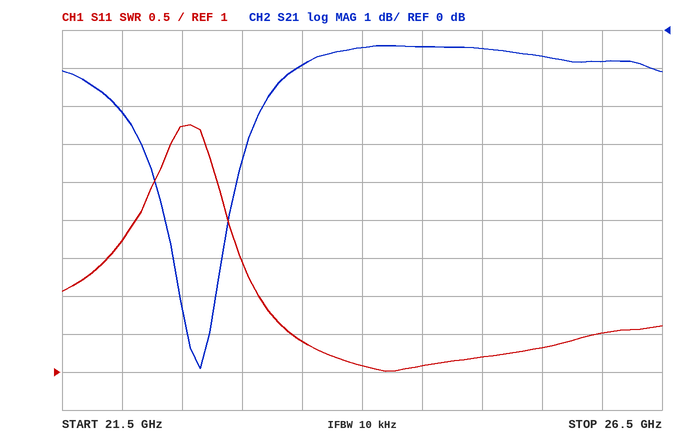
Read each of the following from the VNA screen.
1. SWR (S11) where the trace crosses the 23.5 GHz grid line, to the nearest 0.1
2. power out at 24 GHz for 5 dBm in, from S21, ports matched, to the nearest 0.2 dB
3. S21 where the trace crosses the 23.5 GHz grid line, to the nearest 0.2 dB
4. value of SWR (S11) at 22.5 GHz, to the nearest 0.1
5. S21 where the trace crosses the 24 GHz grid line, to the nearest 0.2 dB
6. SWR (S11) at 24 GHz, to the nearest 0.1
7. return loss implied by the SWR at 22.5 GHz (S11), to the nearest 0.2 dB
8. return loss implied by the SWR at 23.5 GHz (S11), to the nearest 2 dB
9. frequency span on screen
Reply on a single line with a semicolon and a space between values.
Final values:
1.4; 4.6 dBm; -1.0 dB; 4.2; -0.4 dB; 1.1; 4.2 dB; 16 dB; 5 GHz
